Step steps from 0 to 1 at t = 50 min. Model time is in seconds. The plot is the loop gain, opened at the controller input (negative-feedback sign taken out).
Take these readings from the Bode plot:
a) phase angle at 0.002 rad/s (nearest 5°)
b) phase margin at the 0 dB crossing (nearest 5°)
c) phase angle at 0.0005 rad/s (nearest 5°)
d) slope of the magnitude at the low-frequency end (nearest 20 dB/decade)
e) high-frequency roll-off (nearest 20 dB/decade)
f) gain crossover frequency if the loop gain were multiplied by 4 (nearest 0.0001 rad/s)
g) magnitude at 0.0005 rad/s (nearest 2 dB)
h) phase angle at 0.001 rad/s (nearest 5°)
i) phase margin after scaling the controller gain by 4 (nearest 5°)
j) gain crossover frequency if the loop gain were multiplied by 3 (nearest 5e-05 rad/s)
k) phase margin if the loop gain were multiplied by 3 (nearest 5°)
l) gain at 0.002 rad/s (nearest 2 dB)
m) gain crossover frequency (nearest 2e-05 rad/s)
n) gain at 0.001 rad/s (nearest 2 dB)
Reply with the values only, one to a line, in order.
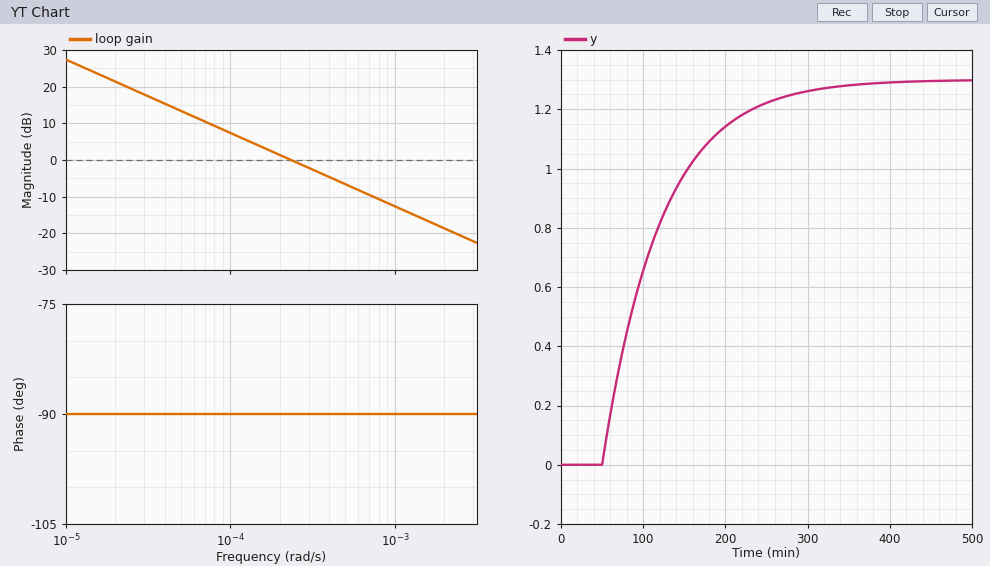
-90°
90°
-90°
-20 dB/decade
-20 dB/decade
0.0009 rad/s
-6 dB
-90°
90°
0.00070 rad/s
90°
-18 dB
0.00024 rad/s
-12 dB
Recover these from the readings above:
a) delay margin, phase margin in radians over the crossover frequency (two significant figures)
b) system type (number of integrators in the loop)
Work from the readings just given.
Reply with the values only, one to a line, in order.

6500 s
1
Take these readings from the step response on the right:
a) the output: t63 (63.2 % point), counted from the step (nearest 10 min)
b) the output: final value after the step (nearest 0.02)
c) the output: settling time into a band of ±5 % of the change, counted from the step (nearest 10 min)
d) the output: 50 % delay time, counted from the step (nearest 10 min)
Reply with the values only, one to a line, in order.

70 min
1.30
210 min
50 min
